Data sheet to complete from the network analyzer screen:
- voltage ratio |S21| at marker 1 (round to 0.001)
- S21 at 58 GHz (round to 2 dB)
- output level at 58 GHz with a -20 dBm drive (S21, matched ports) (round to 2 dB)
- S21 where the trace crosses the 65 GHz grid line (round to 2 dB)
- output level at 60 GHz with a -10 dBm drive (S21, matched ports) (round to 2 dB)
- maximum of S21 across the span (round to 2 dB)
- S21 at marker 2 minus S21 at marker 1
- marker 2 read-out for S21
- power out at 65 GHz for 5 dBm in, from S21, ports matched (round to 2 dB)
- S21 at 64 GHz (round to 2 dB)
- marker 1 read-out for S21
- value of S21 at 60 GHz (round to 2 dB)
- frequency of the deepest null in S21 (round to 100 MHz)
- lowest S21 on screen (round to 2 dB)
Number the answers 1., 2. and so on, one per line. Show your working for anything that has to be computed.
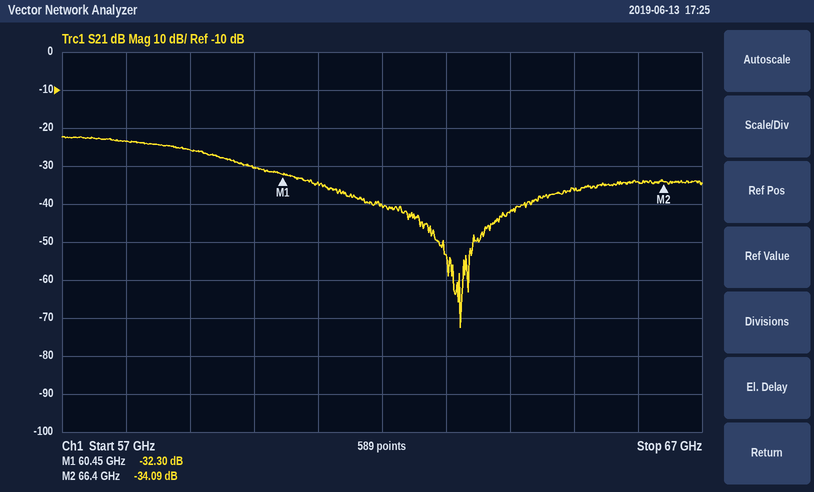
1. 10^(-32.3/20) ≈ 0.024
2. -24 dB
3. -20 dBm + (-24 dB) = -44 dBm
4. -36 dB
5. -10 dBm + (-30 dB) = -40 dBm
6. -22 dB
7. -34.09 − (-32.3) = -1.79 dB
8. -34.09 dB
9. 5 dBm + (-36 dB) = -32 dBm
10. -42 dB
11. -32.30 dB
12. -30 dB
13. 63.2 GHz
14. -72 dB
